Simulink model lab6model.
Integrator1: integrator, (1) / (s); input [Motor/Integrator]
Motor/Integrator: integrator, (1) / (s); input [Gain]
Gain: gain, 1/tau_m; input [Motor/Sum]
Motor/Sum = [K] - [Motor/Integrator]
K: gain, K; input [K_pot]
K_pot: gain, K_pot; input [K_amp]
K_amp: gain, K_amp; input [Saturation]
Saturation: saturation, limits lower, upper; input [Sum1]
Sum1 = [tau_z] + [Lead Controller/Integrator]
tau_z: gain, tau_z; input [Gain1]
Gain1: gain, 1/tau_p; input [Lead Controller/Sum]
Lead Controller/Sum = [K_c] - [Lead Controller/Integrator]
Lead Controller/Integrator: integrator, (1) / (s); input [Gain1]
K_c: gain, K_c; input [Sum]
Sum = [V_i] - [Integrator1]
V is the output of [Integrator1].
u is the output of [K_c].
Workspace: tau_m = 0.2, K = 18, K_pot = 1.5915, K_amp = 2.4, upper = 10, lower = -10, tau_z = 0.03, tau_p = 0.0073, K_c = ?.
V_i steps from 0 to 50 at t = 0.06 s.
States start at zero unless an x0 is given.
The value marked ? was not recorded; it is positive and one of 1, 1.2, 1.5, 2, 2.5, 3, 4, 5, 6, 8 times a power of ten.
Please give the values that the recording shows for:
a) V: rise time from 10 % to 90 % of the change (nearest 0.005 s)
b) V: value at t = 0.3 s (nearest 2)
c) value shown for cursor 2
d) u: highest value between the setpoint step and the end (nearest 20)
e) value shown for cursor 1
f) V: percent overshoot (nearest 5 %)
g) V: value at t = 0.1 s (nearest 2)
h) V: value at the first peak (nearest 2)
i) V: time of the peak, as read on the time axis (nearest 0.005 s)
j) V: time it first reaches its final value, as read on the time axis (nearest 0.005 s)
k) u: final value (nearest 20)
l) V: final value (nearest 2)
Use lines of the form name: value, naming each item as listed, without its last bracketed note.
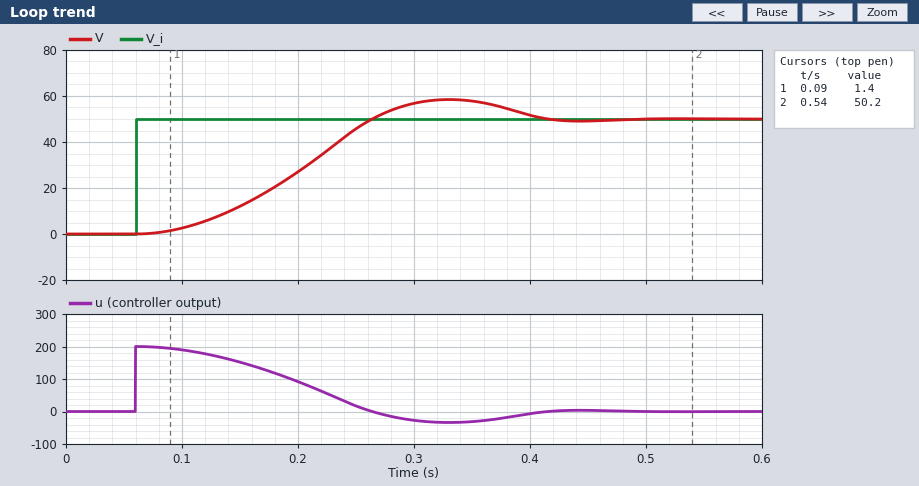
V: rise time from 10 % to 90 % of the change: 0.130 s
V: value at t = 0.3 s: 56
value shown for cursor 2: 50.2
u: highest value between the setpoint step and the end: 200
value shown for cursor 1: 1.4
V: percent overshoot: 15 %
V: value at t = 0.1 s: 2
V: value at the first peak: 58
V: time of the peak, as read on the time axis: 0.330 s
V: time it first reaches its final value, as read on the time axis: 0.265 s
u: final value: 0
V: final value: 50
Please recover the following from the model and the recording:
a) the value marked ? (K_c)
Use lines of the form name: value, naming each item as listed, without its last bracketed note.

the value marked ?: 4
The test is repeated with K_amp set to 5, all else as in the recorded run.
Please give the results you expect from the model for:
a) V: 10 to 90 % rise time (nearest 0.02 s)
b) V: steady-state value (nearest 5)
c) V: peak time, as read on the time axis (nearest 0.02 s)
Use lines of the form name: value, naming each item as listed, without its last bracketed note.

V: 10 to 90 % rise time: 0.08 s
V: steady-state value: 50
V: peak time, as read on the time axis: 0.24 s
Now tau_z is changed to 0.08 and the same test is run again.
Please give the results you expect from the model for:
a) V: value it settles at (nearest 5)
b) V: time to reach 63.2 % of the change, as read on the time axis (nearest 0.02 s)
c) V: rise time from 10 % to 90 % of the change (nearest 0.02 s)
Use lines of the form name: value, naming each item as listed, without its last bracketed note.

V: value it settles at: 50
V: time to reach 63.2 % of the change, as read on the time axis: 0.22 s
V: rise time from 10 % to 90 % of the change: 0.20 s
